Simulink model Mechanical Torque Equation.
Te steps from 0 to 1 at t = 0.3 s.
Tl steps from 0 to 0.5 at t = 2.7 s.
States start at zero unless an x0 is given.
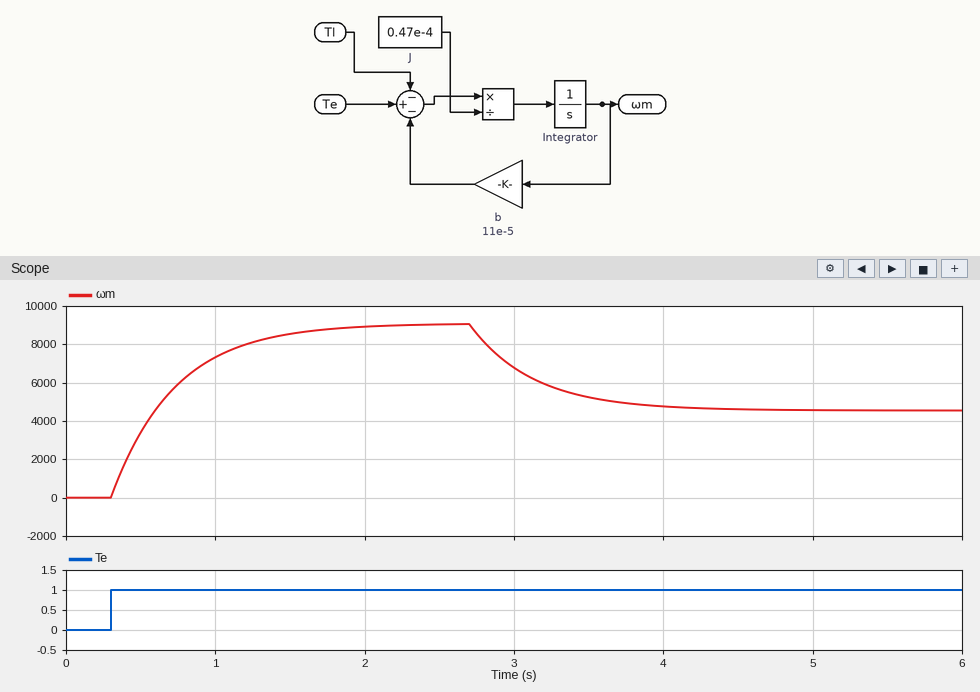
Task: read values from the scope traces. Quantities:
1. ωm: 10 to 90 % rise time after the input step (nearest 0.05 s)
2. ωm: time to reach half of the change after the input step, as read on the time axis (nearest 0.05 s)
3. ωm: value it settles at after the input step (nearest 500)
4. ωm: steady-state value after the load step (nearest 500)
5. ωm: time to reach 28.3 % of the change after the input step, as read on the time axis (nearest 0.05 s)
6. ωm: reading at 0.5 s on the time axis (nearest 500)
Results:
0.95 s
0.60 s
9000
4500
0.45 s
3500
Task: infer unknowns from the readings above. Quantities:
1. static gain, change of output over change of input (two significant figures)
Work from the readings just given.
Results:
9000
